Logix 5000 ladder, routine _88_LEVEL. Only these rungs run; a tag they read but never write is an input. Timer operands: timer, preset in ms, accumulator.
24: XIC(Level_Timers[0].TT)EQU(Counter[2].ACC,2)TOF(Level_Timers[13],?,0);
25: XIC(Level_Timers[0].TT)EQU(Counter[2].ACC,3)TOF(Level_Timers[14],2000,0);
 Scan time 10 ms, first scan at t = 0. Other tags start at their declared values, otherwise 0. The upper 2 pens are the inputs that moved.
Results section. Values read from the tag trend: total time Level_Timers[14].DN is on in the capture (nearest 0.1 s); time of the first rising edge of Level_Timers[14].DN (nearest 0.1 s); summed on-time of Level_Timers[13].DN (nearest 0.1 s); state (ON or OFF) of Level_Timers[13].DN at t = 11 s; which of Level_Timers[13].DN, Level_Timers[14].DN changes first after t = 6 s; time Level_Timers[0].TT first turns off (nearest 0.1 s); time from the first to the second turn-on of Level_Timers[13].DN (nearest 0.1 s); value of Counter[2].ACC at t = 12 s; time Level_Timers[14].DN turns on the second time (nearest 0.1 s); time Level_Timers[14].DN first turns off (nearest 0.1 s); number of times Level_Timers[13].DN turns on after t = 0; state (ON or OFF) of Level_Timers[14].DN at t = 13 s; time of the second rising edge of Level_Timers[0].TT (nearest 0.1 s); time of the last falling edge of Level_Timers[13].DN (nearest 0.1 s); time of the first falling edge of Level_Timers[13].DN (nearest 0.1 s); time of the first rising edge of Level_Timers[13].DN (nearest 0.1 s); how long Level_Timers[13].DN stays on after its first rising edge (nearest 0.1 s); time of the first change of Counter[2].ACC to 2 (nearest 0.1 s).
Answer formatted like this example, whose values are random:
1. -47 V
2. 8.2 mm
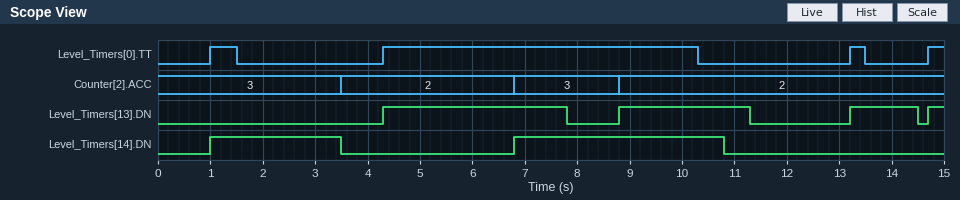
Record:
1. 6.5 s
2. 1.0 s
3. 7.6 s
4. ON
5. Level_Timers[14].DN
6. 1.5 s
7. 4.5 s
8. 2
9. 6.8 s
10. 3.5 s
11. 4
12. OFF
13. 4.3 s
14. 14.5 s
15. 7.8 s
16. 4.3 s
17. 3.5 s
18. 3.5 s
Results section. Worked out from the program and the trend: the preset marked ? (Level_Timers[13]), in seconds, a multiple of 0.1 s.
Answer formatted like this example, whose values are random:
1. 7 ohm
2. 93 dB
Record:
1. 1.0 s
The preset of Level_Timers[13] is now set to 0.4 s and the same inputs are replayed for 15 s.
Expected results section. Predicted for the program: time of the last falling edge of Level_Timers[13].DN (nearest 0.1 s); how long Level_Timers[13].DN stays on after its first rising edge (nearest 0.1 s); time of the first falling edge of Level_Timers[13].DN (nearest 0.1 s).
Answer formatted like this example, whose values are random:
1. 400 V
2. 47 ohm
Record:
1. 13.9 s
2. 2.9 s
3. 7.2 s
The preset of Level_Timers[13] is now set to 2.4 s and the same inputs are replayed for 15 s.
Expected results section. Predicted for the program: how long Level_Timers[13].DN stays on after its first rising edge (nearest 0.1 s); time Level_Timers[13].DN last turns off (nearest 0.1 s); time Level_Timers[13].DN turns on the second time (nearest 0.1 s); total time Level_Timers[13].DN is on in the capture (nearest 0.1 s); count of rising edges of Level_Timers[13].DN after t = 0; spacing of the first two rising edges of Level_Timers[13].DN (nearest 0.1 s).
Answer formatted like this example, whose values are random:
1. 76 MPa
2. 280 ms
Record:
1. 8.4 s
2. 12.7 s
3. 13.2 s
4. 10.2 s
5. 2
6. 8.9 s
